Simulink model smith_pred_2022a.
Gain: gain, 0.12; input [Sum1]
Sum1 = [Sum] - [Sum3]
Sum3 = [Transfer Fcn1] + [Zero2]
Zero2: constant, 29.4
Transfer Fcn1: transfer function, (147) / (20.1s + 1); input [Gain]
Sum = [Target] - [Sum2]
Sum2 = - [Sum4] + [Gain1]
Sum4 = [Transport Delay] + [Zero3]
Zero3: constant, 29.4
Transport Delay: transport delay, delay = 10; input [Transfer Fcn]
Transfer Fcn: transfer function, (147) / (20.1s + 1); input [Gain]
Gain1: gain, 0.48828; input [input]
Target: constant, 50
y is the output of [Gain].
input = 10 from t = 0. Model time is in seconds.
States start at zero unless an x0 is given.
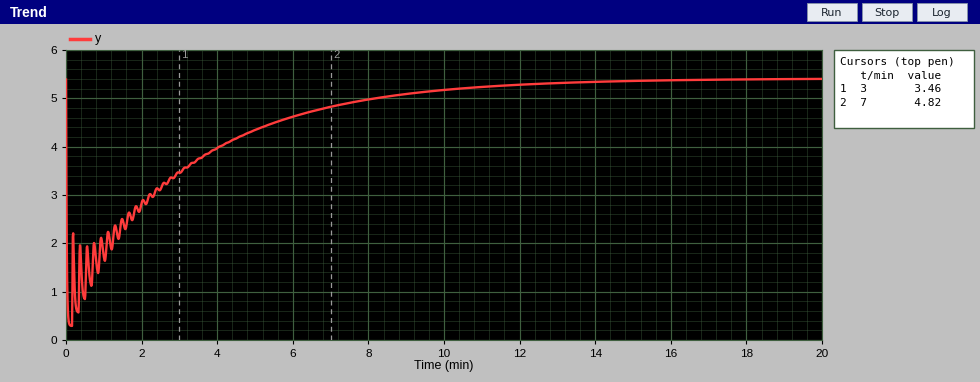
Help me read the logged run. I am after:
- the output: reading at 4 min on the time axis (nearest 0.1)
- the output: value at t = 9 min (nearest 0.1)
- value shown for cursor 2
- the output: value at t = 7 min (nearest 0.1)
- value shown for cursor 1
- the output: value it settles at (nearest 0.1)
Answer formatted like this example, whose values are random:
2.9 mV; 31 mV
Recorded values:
4.0; 5.1; 4.82; 4.8; 3.46; 5.4
